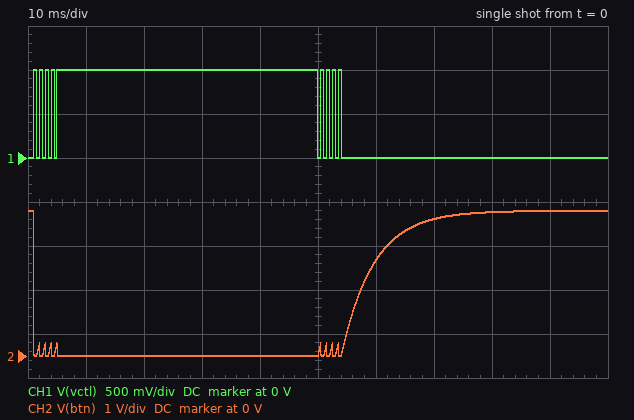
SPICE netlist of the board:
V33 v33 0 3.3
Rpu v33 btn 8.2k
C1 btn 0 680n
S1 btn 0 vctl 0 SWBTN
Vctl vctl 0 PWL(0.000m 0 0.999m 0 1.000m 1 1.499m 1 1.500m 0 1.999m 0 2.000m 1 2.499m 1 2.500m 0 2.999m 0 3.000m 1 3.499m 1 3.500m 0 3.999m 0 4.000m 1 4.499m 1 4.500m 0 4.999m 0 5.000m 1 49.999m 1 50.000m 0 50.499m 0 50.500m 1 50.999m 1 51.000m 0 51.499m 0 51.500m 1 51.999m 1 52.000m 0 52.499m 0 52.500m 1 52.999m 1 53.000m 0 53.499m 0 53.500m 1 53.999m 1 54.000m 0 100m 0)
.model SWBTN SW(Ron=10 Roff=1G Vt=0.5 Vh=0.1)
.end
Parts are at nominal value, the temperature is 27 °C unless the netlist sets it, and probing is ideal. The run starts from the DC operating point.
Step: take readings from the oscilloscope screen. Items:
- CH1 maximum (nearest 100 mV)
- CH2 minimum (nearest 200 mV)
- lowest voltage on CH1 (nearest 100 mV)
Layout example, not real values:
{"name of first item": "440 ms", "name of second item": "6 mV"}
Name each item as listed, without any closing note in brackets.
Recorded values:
{"CH1 maximum": "1.0 V", "CH2 minimum": "0 V", "lowest voltage on CH1": "0 V"}
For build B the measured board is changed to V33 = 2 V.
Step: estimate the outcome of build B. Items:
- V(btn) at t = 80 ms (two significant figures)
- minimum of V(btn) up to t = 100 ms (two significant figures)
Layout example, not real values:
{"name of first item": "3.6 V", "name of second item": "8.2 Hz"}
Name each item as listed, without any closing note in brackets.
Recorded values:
{"V(btn) at t = 80 ms": "2.0 V", "minimum of V(btn) up to t = 100 ms": "2.4 mV"}
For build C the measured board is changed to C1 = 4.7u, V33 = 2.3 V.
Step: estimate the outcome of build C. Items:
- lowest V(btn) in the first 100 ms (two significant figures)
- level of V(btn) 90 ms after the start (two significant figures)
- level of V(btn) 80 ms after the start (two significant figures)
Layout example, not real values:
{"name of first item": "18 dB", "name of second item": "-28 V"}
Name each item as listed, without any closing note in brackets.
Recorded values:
{"lowest V(btn) in the first 100 ms": "2.8 mV", "level of V(btn) 90 ms after the start": "1.4 V", "level of V(btn) 80 ms after the start": "1.1 V"}
